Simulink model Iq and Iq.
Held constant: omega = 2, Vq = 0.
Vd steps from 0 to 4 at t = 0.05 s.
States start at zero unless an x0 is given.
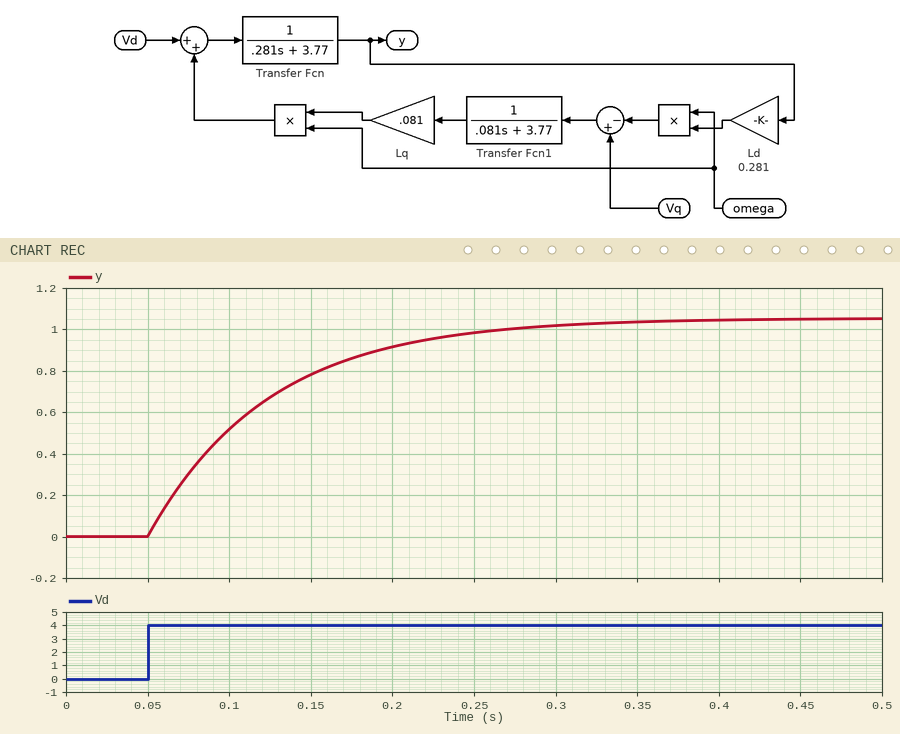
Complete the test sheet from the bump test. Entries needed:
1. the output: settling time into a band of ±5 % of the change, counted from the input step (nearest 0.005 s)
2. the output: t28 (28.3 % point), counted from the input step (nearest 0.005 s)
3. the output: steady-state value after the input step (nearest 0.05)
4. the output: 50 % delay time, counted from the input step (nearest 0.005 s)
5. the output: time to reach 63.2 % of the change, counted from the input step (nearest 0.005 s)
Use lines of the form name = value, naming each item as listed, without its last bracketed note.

the output: settling time into a band of ±5 % of the change, counted from the input step = 0.220 s
the output: t28 (28.3 % point), counted from the input step = 0.025 s
the output: steady-state value after the input step = 1.05
the output: 50 % delay time, counted from the input step = 0.050 s
the output: time to reach 63.2 % of the change, counted from the input step = 0.075 s
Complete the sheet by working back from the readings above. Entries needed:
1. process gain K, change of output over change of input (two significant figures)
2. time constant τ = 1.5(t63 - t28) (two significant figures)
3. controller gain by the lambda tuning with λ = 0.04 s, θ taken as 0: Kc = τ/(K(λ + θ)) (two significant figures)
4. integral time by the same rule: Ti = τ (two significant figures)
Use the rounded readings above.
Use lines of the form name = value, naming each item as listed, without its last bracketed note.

process gain K, change of output over change of input = 0.26
time constant τ = 1.5(t63 - t28) = 0.075 s
controller gain by the lambda tuning with λ = 0.04 s, θ taken as 0: Kc = τ/(K(λ + θ)) = 7.2
integral time by the same rule: Ti = τ = 0.075 s
